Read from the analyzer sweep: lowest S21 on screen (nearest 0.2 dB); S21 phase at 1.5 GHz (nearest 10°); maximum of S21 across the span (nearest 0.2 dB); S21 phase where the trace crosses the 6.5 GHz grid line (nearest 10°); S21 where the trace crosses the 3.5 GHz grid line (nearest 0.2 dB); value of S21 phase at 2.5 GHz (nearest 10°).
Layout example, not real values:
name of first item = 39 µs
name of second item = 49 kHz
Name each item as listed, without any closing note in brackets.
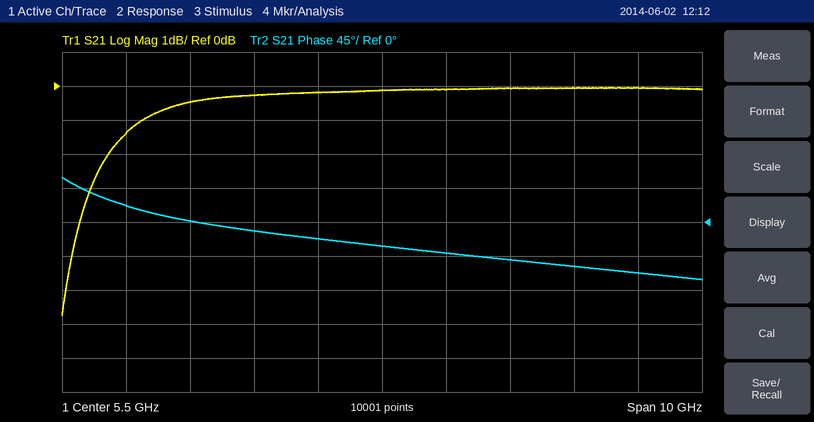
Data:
lowest S21 on screen = -6.8 dB
S21 phase at 1.5 GHz = 20°
maximum of S21 across the span = 0.0 dB
S21 phase where the trace crosses the 6.5 GHz grid line = -40°
S21 where the trace crosses the 3.5 GHz grid line = -0.2 dB
value of S21 phase at 2.5 GHz = 0°
